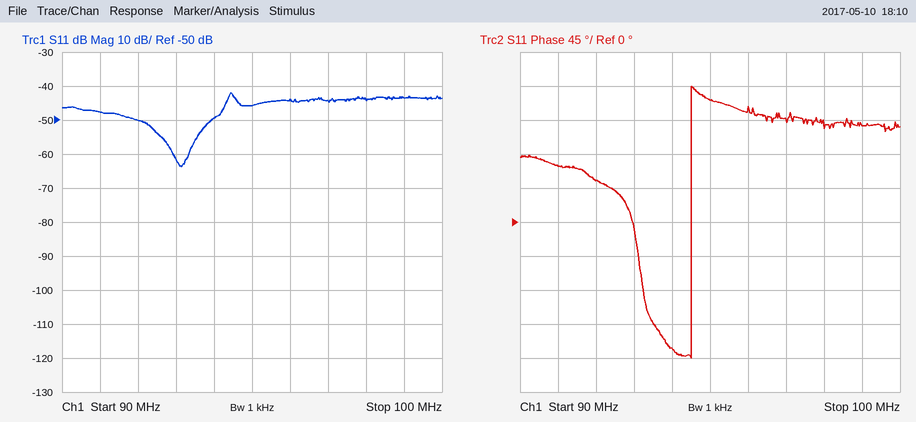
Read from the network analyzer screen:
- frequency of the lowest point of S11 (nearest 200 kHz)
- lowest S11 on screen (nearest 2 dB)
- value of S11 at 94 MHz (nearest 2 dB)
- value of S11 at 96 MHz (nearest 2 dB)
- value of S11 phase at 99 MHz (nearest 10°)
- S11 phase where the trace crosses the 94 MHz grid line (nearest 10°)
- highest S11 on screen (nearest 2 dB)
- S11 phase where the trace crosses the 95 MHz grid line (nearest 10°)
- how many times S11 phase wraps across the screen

93.2 MHz
-64 dB
-50 dB
-44 dB
130°
-170°
-42 dB
160°
1
